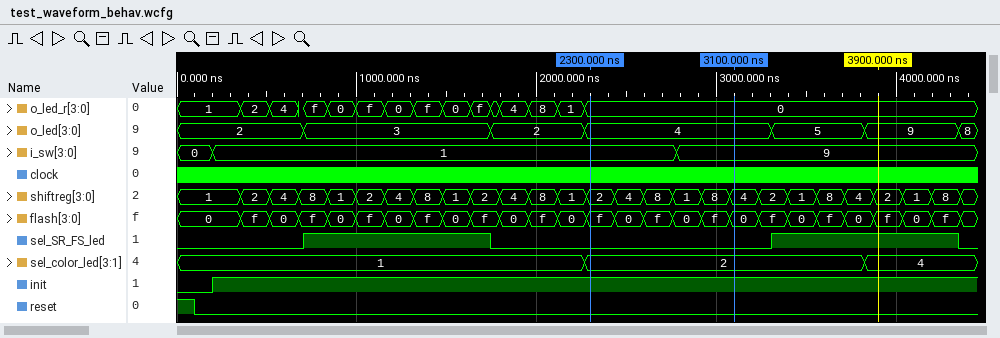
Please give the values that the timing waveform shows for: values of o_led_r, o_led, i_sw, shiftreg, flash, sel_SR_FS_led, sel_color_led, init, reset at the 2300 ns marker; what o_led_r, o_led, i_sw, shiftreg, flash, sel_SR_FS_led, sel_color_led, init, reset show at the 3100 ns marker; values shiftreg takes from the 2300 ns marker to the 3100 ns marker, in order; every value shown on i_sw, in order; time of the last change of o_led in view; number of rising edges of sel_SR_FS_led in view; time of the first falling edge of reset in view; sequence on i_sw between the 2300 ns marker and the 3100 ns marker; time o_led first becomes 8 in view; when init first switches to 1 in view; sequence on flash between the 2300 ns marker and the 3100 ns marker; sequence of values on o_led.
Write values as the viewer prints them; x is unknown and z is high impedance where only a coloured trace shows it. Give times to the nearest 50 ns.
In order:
o_led_r=0, o_led=4, i_sw=1, shiftreg=2, flash=f, sel_SR_FS_led=0, sel_color_led=2, init=1, reset=0
o_led_r=0, o_led=4, i_sw=9, shiftreg=4, flash=0, sel_SR_FS_led=0, sel_color_led=2, init=1, reset=0
2, 4, 8, 1, 8, 4
0, 1, 9
4350 ns
2
100 ns
1, 9
4350 ns
200 ns
f, 0, f, 0, f, 0
2, 3, 2, 4, 5, 9, 8
